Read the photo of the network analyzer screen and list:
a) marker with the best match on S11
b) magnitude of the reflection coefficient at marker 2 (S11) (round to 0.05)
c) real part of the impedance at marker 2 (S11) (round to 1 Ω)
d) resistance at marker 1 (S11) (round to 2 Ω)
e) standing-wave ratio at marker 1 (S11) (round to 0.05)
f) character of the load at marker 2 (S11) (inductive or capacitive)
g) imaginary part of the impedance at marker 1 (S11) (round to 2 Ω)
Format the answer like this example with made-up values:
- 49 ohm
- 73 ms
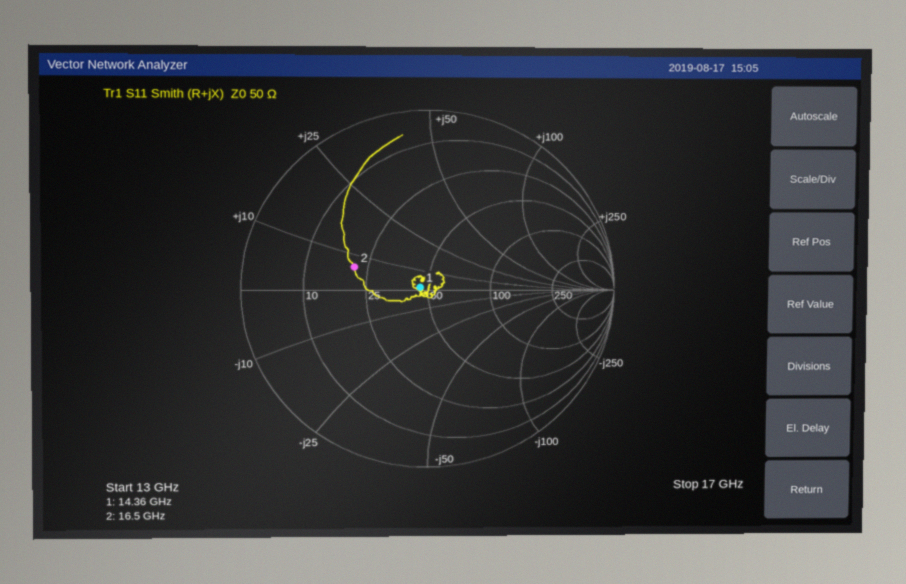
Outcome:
- marker 1
- 0.40
- 21 Ω
- 46 Ω
- 1.10
- inductive
- +2 Ω
